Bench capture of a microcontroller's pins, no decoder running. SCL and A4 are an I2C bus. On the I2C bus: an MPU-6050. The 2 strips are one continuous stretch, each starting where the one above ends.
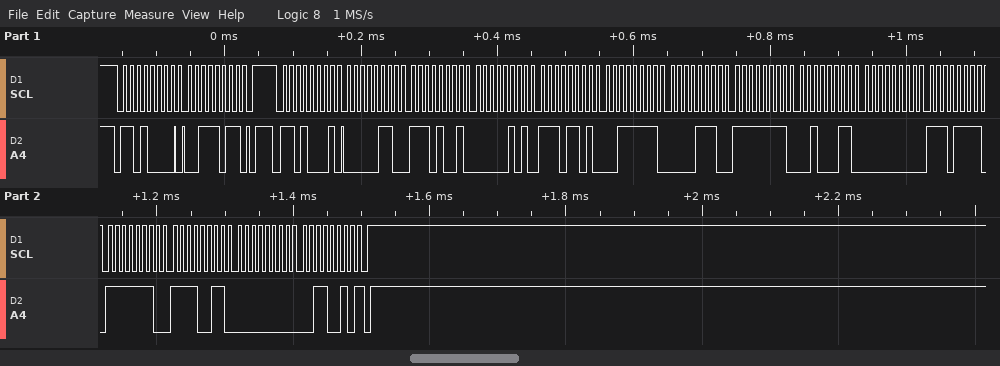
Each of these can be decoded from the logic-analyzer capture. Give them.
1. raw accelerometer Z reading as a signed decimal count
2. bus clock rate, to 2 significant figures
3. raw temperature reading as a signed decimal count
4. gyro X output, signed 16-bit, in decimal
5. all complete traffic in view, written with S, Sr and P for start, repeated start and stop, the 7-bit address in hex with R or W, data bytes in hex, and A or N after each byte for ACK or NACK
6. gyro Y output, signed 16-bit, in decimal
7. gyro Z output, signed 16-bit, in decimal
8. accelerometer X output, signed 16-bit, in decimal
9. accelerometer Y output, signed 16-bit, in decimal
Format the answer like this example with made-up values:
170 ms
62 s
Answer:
16142
100 kHz
-221
239
S 68W A 3B A P S 68R A 06 A E9 A 05 A ED A 3F A 0E A FF A 23 A 00 A EF A FE A F3 A 00 A 32 N P
-269
50
1769
1517
